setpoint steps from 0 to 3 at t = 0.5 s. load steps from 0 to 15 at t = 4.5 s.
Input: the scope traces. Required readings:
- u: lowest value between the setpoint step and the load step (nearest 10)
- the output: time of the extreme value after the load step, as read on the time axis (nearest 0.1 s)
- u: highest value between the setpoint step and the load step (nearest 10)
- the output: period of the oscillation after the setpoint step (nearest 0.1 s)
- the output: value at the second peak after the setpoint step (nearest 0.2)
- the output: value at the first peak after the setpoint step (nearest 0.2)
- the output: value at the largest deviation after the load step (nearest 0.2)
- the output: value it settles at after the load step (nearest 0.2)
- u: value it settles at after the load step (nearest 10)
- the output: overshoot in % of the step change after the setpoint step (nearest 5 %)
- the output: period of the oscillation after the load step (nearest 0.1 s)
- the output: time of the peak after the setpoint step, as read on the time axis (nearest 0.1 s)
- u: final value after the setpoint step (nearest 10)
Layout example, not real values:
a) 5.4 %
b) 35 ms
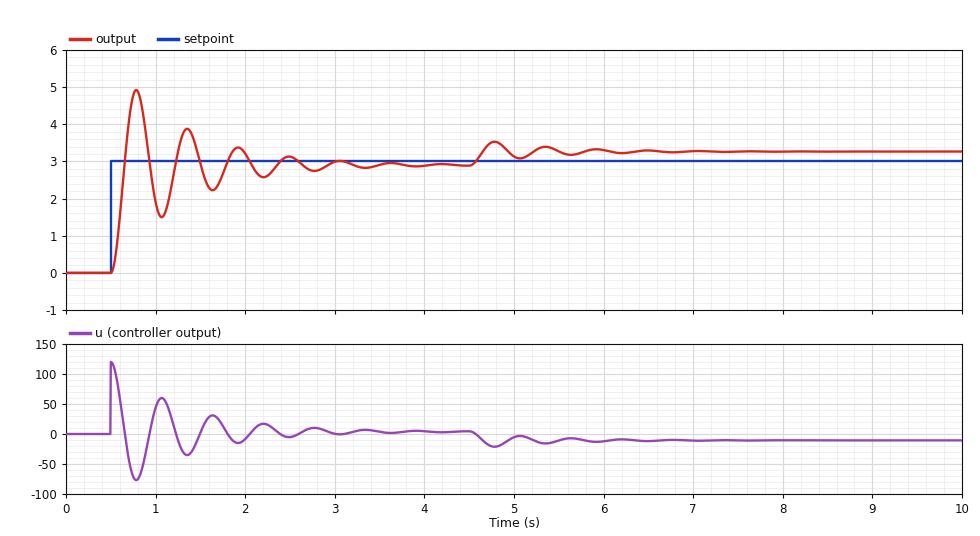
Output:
a) -80
b) 4.8 s
c) 120
d) 0.6 s
e) 3.8
f) 5.0
g) 3.6
h) 3.2
i) -10
j) 70 %
k) 0.6 s
l) 0.8 s
m) 0
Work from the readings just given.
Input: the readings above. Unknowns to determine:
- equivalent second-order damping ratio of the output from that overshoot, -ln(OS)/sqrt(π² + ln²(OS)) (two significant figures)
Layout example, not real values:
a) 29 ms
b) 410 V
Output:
a) 0.11
